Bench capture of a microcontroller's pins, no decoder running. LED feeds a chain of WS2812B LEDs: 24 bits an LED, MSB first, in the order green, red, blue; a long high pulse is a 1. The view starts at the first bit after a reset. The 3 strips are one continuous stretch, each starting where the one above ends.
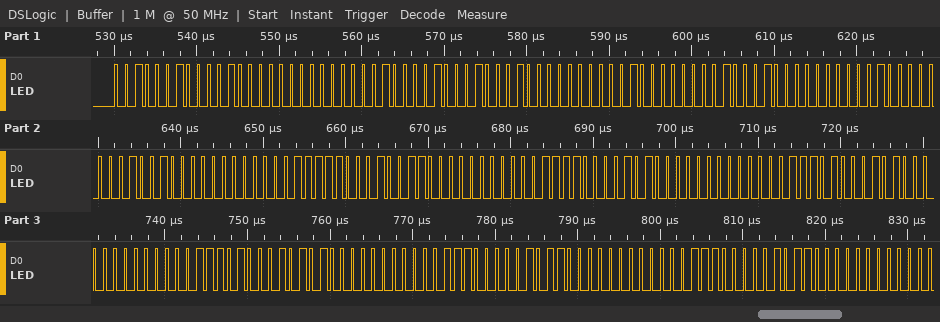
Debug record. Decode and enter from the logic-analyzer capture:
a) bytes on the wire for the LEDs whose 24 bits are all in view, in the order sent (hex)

22 10 00 21 11 00 20 11 00 20 12 00 1F 13 00 1E 14 00 1D 14 00 1D 15 00 1C 16 00 1C 16 00
